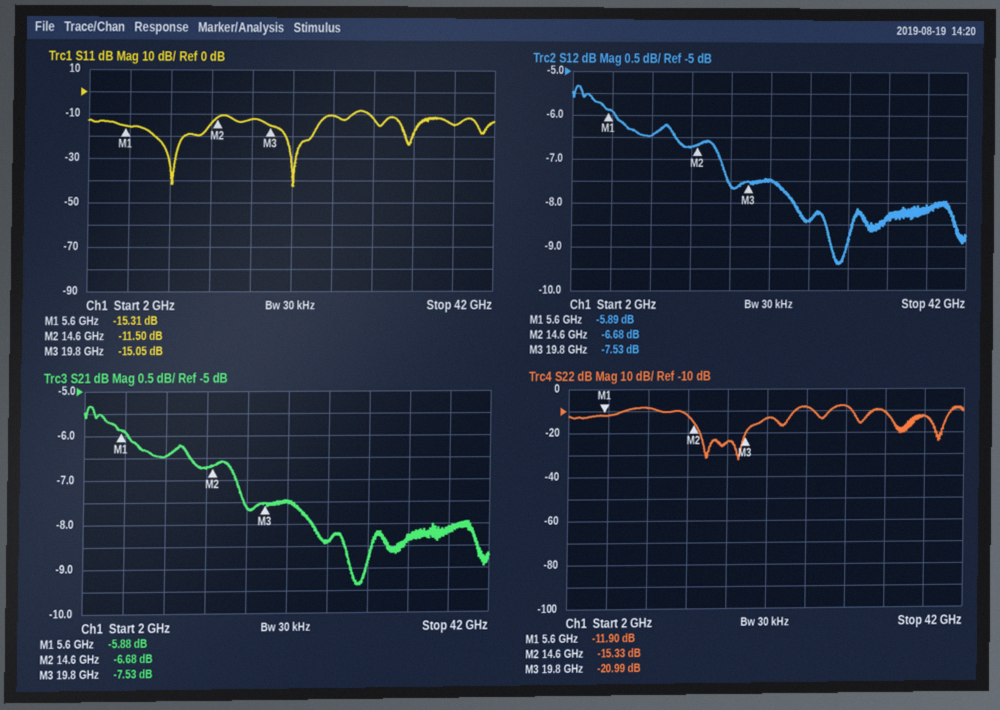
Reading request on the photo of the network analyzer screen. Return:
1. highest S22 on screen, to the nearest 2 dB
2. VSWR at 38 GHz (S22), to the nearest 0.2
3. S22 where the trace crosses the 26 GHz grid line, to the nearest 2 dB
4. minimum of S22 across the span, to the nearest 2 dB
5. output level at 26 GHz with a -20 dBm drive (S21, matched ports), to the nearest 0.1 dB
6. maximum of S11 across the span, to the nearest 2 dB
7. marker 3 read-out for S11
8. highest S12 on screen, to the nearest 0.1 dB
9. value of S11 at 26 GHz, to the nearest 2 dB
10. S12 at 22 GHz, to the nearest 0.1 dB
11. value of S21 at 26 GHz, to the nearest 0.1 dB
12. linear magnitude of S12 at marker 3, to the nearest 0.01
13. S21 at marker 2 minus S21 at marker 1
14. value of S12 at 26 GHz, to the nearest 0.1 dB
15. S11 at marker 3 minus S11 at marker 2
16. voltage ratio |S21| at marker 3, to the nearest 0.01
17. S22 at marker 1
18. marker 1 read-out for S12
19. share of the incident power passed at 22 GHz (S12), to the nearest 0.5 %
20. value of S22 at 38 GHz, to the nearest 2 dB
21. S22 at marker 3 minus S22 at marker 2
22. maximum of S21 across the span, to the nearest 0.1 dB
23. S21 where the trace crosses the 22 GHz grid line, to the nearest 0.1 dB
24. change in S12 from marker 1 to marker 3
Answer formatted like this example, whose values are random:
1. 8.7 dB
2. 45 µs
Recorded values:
1. -8 dB
2. 1.6
3. -8 dB
4. -32 dB
5. -28.4 dBm
6. -8 dB
7. -15.05 dB
8. -5.3 dB
9. -10 dB
10. -7.5 dB
11. -8.4 dB
12. 0.42
13. -0.80 dB
14. -8.4 dB
15. -3.55 dB
16. 0.42
17. -11.90 dB
18. -5.89 dB
19. 18.0 %
20. -12 dB
21. -5.66 dB
22. -5.3 dB
23. -7.5 dB
24. -1.64 dB
